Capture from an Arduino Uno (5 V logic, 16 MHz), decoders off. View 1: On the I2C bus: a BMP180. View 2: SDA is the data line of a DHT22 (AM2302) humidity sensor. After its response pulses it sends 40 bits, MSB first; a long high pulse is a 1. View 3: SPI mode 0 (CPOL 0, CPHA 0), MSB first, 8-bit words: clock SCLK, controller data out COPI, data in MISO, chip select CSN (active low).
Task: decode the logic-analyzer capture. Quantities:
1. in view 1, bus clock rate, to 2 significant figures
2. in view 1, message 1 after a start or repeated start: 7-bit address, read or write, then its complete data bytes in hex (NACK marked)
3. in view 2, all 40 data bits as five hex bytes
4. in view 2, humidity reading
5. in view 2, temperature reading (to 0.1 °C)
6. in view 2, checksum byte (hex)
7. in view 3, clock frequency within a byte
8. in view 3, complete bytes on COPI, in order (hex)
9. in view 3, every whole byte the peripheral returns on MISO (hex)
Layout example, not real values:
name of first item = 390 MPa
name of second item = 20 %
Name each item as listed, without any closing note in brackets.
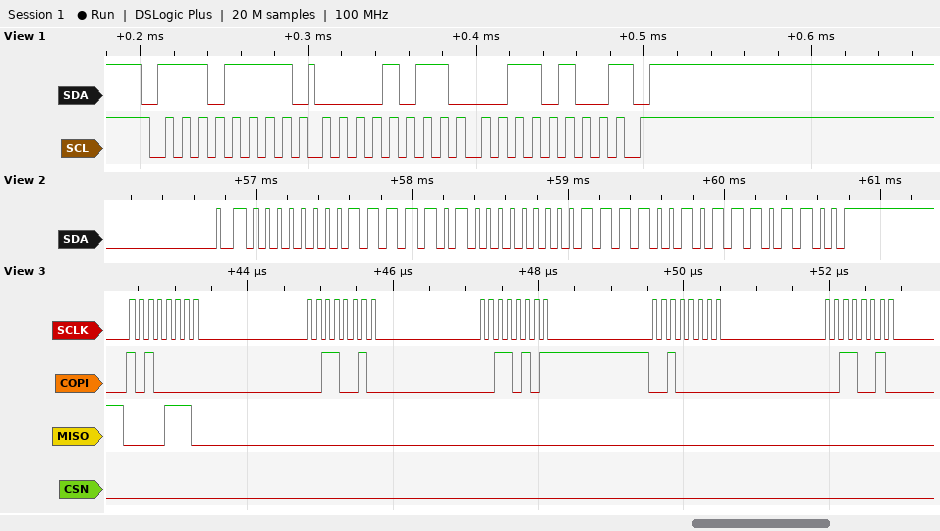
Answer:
in view 1, bus clock rate, to 2 significant figures = 100 kHz
in view 1, message 1 after a start or repeated start: 7-bit address, read or write, then its complete data bytes in hex = 0x77 read: 0B 34 NACK
in view 2, all 40 data bits as five hex bytes = 00 FA 00 F2 EC
in view 2, humidity reading = 25.0 %
in view 2, temperature reading = 24.2 °C
in view 2, checksum byte = 0xEC
in view 3, clock frequency within a byte = 8 MHz
in view 3, complete bytes on COPI, in order = A0 32 35 20 32
in view 3, every whole byte the peripheral returns on MISO = 0E 00 00 00 00
